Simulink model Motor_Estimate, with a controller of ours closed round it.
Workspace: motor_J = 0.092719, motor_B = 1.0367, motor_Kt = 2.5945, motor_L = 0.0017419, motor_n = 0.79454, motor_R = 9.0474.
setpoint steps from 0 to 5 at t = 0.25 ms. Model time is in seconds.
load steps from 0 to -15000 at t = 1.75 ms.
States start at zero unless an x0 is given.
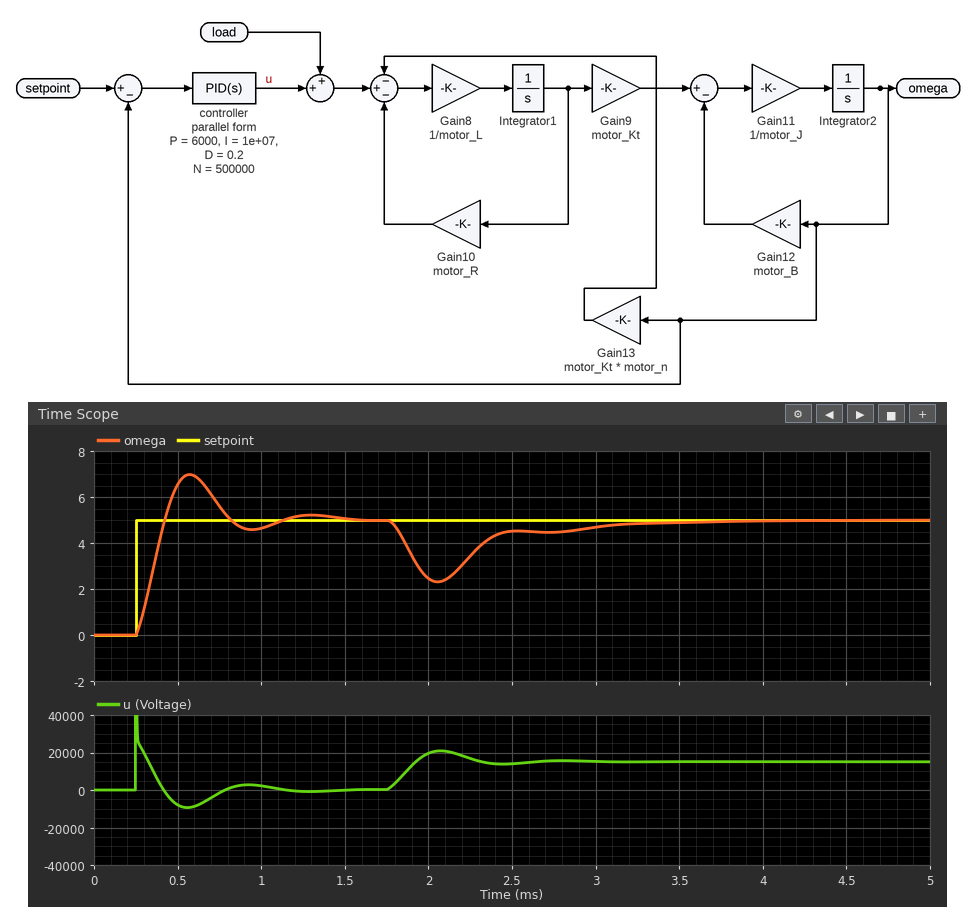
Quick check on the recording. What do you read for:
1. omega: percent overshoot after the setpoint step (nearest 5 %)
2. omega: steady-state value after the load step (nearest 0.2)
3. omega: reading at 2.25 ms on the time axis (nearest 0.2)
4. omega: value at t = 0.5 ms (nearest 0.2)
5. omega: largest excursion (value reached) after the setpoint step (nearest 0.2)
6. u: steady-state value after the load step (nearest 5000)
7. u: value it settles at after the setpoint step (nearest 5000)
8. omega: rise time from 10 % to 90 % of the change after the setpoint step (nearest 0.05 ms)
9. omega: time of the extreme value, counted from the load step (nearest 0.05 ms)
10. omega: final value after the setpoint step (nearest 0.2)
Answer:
40 %
5.0
3.4
6.6
7.0
15000
0
0.15 ms
0.30 ms
5.0
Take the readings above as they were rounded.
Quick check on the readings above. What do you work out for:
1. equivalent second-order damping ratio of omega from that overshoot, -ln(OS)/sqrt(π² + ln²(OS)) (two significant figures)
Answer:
0.28
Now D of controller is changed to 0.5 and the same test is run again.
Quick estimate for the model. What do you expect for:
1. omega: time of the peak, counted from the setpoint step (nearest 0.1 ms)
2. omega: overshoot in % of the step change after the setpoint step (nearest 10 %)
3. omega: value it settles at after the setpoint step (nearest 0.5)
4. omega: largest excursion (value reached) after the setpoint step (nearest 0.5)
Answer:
0.3 ms
20 %
5.0
6.0
